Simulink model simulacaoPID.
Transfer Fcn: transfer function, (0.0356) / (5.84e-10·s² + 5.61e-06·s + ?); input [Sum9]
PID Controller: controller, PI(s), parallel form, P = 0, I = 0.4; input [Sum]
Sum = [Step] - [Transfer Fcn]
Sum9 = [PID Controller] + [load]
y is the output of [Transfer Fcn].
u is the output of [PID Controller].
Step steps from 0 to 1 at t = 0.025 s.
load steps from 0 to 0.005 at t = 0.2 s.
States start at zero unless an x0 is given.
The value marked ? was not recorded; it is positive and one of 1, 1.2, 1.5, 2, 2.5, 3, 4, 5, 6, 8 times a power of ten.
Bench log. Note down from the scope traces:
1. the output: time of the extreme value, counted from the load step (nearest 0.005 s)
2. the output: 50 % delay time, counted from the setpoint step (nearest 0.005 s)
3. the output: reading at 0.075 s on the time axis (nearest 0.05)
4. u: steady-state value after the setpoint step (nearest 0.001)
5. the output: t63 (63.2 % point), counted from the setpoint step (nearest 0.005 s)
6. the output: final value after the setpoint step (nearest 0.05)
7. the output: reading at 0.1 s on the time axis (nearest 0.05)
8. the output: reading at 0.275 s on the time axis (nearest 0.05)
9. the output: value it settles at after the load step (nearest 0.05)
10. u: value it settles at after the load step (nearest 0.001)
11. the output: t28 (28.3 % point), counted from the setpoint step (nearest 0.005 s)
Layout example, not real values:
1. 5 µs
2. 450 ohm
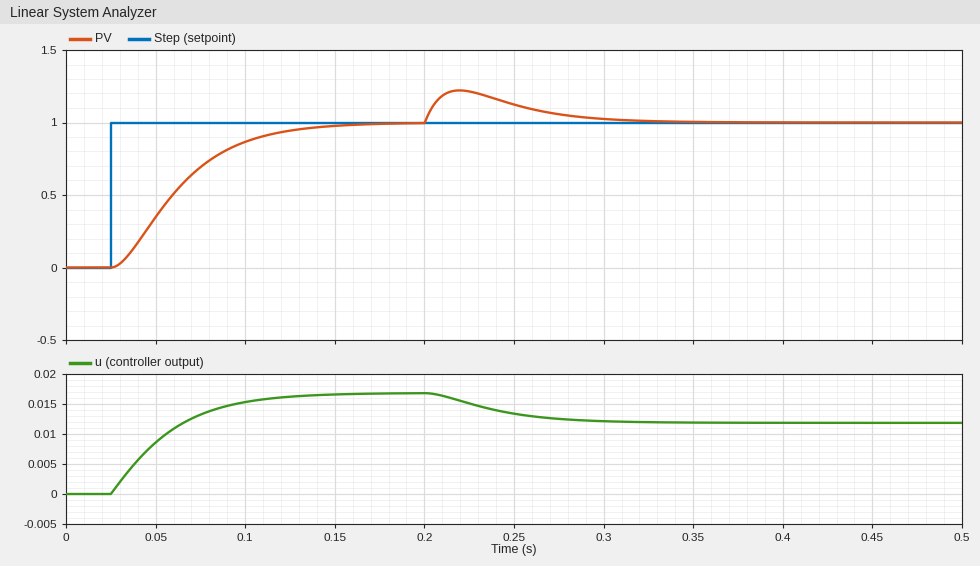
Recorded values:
1. 0.020 s
2. 0.035 s
3. 0.70
4. 0.017
5. 0.045 s
6. 1.00
7. 0.85
8. 1.05
9. 1.00
10. 0.012
11. 0.020 s
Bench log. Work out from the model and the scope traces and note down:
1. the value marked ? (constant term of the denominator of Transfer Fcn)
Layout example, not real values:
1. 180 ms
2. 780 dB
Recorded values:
1. 0.0006
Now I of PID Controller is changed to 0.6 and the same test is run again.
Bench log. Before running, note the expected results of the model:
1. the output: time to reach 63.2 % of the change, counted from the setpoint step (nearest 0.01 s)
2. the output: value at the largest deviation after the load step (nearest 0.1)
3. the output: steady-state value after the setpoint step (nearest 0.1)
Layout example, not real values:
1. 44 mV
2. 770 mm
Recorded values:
1. 0.03 s
2. 1.2
3. 1.0
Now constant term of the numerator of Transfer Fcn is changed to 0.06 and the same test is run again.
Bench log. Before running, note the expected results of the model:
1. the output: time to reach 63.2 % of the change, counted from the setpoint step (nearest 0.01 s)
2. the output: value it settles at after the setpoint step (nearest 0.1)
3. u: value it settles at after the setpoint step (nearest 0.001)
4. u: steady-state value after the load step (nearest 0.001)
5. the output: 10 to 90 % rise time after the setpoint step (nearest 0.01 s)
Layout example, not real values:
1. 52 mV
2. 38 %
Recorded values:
1. 0.03 s
2. 1.0
3. 0.010
4. 0.005
5. 0.04 s
